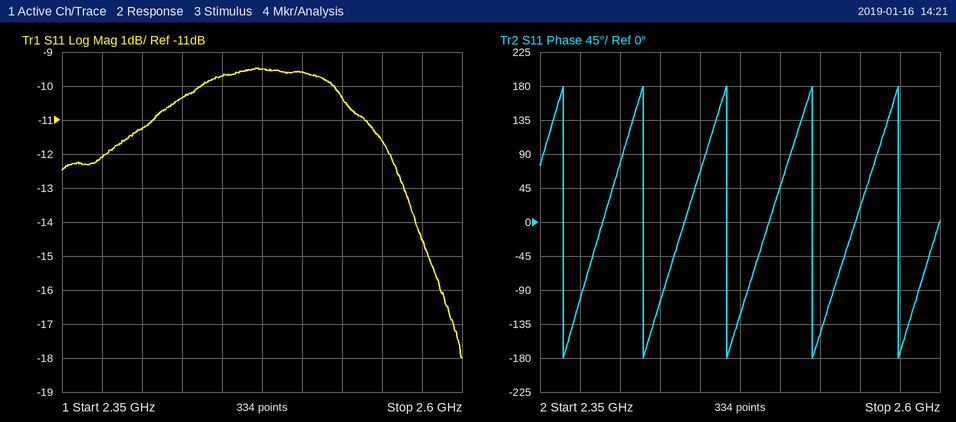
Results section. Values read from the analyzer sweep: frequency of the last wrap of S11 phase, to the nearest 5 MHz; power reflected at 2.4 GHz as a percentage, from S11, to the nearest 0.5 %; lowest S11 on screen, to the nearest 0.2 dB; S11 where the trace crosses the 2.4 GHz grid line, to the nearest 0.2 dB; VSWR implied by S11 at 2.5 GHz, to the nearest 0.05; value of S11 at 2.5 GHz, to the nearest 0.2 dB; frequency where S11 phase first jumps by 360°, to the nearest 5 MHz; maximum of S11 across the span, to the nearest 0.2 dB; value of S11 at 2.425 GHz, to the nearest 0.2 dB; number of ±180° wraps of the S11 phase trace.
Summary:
2.575 GHz
7.5 %
-18.0 dB
-11.2 dB
2.00
-9.6 dB
2.365 GHz
-9.4 dB
-10.4 dB
5
